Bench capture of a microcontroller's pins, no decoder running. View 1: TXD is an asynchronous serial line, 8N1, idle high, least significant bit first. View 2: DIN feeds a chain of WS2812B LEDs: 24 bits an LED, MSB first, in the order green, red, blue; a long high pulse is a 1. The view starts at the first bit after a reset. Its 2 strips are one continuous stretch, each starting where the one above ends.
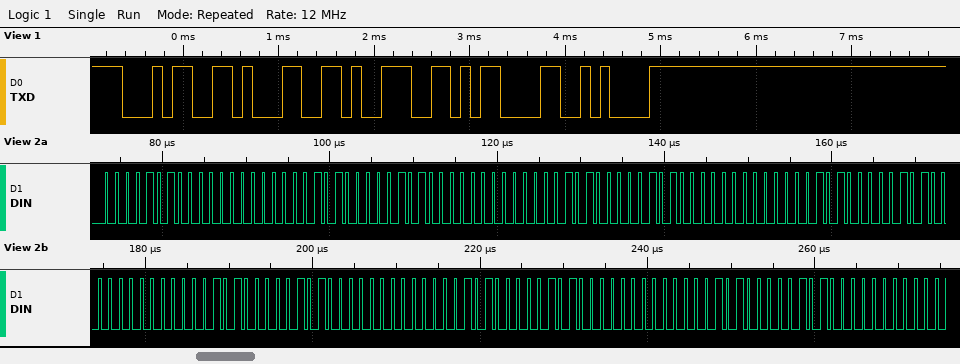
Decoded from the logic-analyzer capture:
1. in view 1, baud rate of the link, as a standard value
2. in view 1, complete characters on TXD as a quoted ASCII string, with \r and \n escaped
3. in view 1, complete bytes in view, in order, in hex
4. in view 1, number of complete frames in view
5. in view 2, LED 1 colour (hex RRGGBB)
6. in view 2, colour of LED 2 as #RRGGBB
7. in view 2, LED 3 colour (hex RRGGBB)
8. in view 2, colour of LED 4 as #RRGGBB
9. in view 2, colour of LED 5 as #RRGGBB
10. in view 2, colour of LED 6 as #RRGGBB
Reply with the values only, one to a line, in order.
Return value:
9600 baud
"419\r\n"
0x34 0x31 0x39 0x0D 0x0A
5
#000A0A
#000A0A
#000A0A
#000A0A
#000A0A
#000A0A
